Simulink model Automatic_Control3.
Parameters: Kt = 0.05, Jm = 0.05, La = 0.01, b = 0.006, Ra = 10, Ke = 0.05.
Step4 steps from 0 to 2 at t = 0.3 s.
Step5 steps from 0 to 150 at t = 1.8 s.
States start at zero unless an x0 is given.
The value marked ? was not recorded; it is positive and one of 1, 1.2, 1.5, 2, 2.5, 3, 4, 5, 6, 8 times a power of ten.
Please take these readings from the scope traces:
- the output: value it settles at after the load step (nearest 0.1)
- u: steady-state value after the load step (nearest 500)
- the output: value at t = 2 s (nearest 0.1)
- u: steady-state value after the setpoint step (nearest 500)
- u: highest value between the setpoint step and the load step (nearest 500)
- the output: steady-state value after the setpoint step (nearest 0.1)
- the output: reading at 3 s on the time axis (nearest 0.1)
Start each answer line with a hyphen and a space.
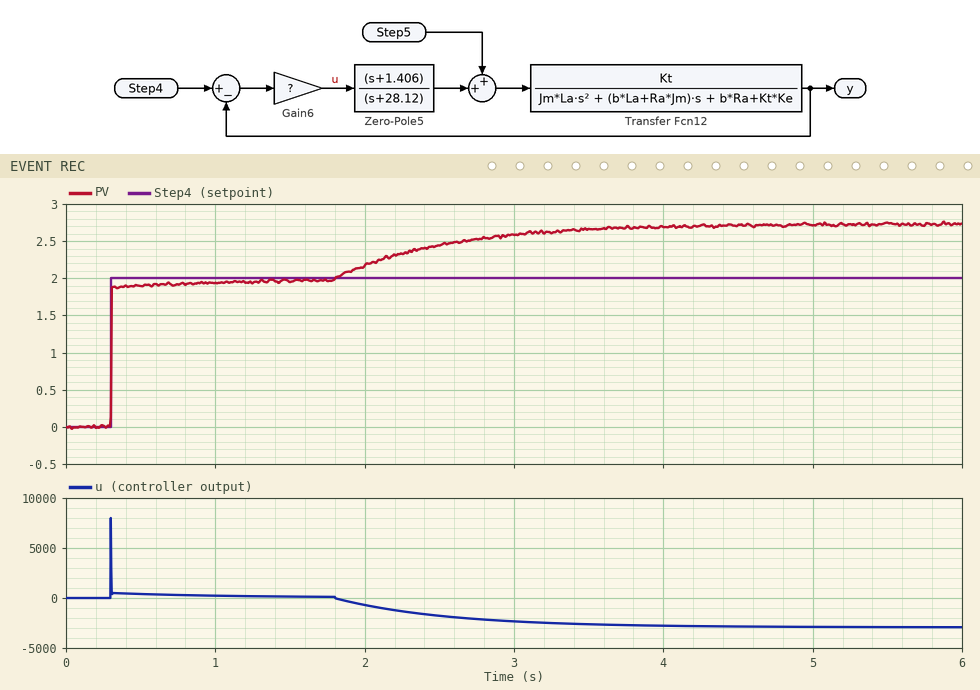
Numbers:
- 2.7
- -3000
- 2.2
- 0
- 8000
- 2.0
- 2.6
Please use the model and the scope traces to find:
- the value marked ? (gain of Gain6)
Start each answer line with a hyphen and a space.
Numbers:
- 4000
